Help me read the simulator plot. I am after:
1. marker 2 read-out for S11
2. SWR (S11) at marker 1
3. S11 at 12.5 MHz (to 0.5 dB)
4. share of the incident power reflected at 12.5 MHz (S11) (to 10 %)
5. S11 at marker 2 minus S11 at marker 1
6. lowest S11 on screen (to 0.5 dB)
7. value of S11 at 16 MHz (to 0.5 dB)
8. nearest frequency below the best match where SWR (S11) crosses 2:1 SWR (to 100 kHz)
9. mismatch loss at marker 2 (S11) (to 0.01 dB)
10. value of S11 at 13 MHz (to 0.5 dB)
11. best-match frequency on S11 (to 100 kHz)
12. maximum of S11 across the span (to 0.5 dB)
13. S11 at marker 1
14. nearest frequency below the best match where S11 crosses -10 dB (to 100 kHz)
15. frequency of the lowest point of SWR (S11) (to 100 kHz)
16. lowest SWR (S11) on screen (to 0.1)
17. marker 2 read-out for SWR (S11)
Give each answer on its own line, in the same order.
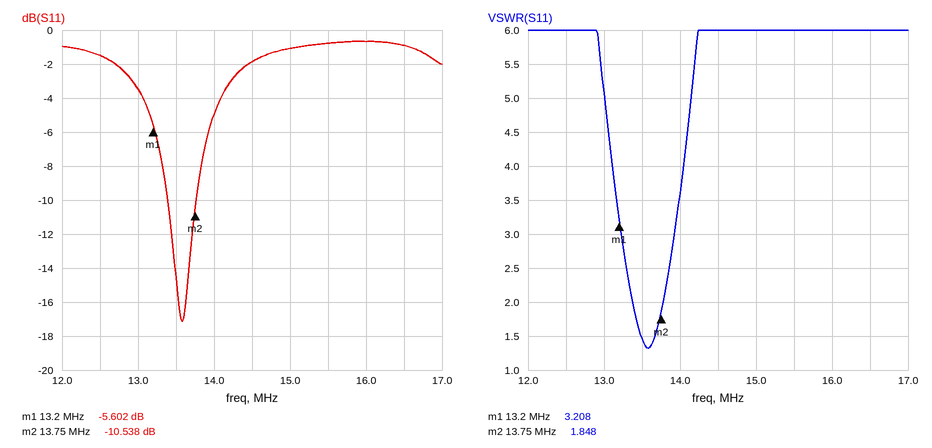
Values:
-10.538 dB
3.208
-1.5 dB
70 %
-4.936 dB
-17.0 dB
-0.5 dB
13.4 MHz
0.40 dB
-3.5 dB
13.6 MHz
-0.5 dB
-5.602 dB
13.4 MHz
13.6 MHz
1.3
1.848
